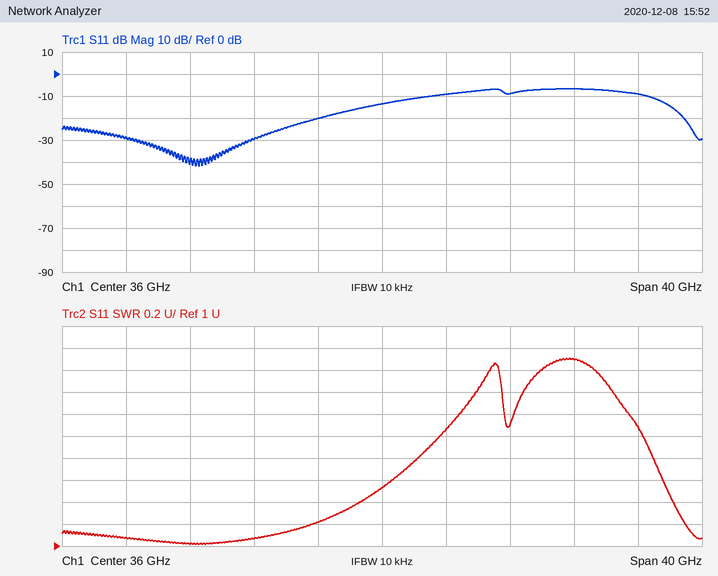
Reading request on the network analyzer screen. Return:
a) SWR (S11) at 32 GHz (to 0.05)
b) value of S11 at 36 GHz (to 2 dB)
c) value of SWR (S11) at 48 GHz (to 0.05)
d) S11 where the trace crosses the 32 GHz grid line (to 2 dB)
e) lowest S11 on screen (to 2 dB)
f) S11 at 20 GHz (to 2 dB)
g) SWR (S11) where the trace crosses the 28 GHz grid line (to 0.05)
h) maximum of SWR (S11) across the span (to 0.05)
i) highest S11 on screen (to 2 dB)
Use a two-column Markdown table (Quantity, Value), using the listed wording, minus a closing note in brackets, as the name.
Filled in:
| Quantity | Value |
|---|---|
| SWR (S11) at 32 GHz | 1.20 |
| value of S11 at 36 GHz | -14 dB |
| value of SWR (S11) at 48 GHz | 2.70 |
| S11 where the trace crosses the 32 GHz grid line | -20 dB |
| lowest S11 on screen | -42 dB |
| S11 at 20 GHz | -28 dB |
| SWR (S11) where the trace crosses the 28 GHz grid line | 1.05 |
| maximum of SWR (S11) across the span | 2.70 |
| highest S11 on screen | -6 dB |
